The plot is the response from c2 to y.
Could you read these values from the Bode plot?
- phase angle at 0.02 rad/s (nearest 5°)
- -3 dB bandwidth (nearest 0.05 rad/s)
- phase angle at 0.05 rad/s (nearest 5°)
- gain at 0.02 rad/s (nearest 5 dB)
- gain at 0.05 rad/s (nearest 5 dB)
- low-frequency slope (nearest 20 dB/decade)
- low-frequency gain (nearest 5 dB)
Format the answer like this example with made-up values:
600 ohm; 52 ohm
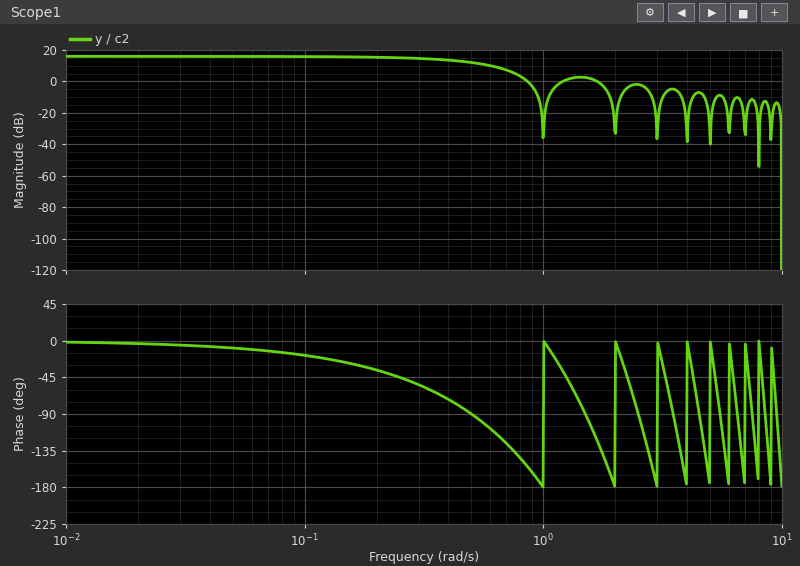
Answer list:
-5°; 0.45 rad/s; -10°; 15 dB; 15 dB; 0 dB/decade; 15 dB
